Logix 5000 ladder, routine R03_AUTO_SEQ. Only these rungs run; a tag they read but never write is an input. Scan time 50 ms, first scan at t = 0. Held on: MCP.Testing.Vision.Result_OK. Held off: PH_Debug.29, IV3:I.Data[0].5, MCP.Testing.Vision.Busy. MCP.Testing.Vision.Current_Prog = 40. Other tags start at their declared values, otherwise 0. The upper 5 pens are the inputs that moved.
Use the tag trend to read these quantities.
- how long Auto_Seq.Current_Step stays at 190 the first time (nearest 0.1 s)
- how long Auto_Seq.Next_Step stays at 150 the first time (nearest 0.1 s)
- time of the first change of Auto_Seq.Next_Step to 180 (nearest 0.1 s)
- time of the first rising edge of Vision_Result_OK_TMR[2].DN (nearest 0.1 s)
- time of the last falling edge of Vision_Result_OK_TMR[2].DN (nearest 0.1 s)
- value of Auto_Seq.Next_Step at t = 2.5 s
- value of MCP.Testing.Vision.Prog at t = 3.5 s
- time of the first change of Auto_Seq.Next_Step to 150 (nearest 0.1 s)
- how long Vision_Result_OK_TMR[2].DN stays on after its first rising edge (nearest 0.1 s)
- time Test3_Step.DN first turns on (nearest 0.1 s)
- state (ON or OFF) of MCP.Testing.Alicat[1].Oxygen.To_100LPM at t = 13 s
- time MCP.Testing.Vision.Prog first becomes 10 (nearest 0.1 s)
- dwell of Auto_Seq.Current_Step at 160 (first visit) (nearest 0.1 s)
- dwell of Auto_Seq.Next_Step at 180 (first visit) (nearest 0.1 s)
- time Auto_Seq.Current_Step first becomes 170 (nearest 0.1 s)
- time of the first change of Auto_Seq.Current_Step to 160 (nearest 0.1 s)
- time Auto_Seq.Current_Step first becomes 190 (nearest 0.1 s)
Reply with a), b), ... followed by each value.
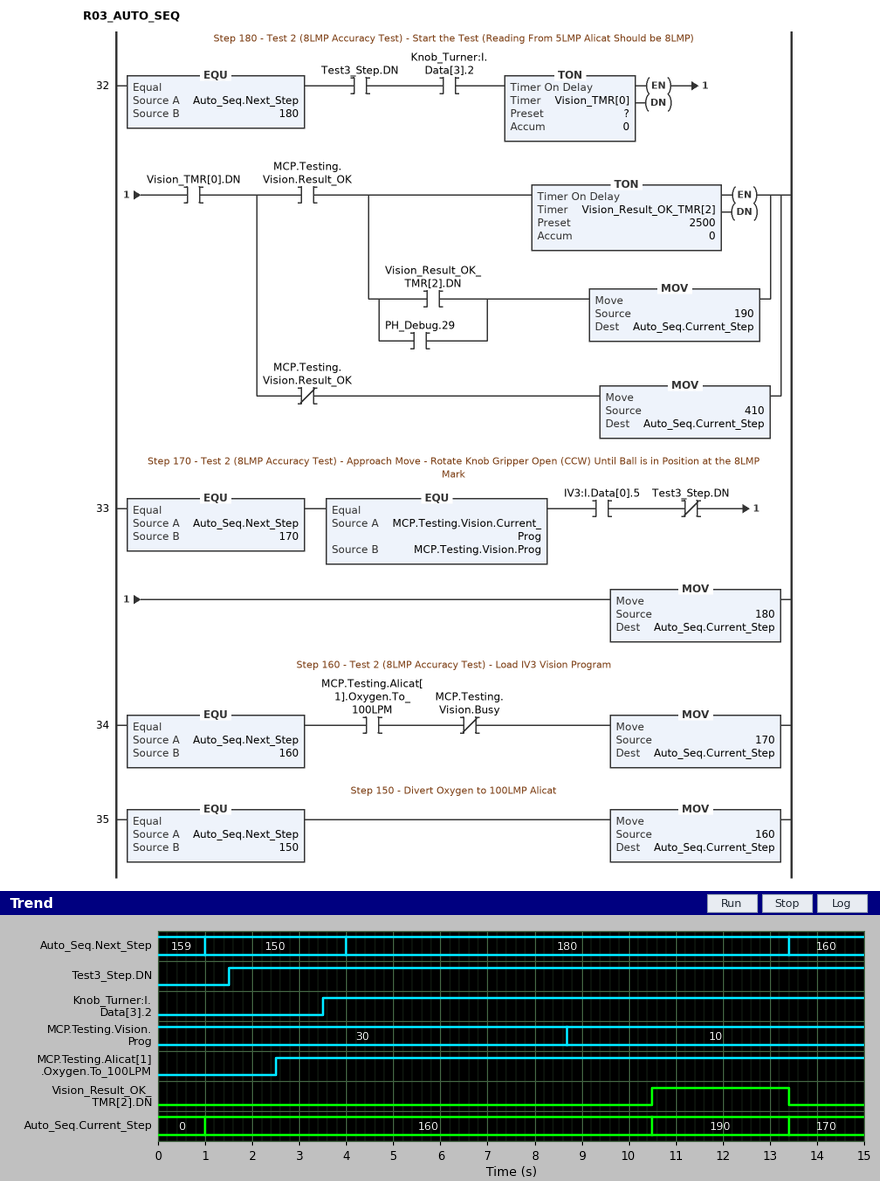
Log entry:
a) 2.9 s
b) 3.0 s
c) 4.0 s
d) 10.5 s
e) 13.4 s
f) 150
g) 30
h) 1.0 s
i) 2.9 s
j) 1.5 s
k) ON
l) 8.7 s
m) 9.5 s
n) 9.4 s
o) 13.4 s
p) 1.0 s
q) 10.5 s
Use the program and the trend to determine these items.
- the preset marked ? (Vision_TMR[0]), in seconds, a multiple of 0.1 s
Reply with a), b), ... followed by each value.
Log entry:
a) 4.0 s
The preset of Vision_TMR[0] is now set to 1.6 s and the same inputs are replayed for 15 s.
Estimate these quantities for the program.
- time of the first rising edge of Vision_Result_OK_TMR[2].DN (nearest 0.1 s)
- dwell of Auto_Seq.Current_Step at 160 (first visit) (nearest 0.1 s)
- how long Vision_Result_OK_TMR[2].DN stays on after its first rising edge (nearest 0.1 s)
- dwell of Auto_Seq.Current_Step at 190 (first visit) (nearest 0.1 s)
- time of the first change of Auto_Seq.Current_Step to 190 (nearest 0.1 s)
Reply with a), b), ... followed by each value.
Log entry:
a) 8.1 s
b) 7.1 s
c) 5.3 s
d) 5.3 s
e) 8.1 s
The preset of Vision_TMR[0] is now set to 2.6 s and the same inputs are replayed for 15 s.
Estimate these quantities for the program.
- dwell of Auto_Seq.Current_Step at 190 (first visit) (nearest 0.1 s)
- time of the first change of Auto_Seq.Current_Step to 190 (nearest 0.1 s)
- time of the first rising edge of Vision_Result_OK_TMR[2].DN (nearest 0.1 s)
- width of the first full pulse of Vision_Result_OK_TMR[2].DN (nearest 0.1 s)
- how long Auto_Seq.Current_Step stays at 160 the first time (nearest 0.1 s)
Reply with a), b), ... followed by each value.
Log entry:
a) 4.3 s
b) 9.1 s
c) 9.1 s
d) 4.3 s
e) 8.1 s
